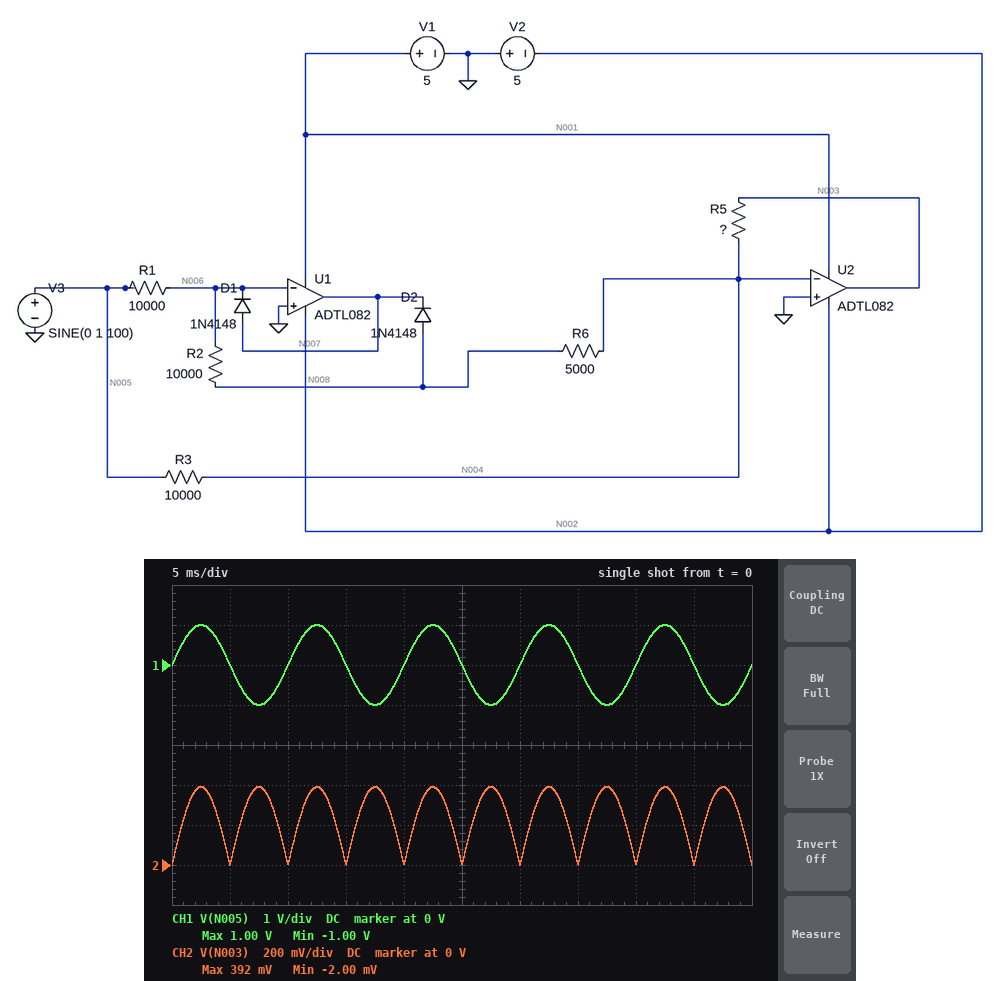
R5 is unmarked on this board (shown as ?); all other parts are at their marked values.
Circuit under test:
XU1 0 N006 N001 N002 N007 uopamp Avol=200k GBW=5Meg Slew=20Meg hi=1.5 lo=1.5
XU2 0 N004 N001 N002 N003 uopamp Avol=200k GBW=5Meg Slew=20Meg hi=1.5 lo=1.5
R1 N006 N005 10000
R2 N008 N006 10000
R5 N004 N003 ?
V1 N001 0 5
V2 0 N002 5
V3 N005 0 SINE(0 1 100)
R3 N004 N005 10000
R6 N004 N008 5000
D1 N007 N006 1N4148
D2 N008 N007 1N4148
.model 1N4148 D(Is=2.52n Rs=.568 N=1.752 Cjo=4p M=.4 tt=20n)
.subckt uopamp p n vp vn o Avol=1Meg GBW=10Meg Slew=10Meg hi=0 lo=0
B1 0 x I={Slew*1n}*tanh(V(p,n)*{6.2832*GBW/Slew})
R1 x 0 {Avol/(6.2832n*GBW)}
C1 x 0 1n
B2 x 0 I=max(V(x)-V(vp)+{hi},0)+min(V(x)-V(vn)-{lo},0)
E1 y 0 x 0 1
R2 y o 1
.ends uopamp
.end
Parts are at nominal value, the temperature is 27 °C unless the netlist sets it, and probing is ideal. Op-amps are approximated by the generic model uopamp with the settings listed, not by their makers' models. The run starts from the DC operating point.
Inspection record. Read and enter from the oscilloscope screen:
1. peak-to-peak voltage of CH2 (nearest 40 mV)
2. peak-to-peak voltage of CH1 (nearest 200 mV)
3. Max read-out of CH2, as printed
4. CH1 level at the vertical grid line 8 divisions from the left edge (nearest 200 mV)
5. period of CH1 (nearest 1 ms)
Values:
400 mV
2.0 V
392 mV
0 V
10 ms
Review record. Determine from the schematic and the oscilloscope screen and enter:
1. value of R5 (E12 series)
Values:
3.9 kΩ
